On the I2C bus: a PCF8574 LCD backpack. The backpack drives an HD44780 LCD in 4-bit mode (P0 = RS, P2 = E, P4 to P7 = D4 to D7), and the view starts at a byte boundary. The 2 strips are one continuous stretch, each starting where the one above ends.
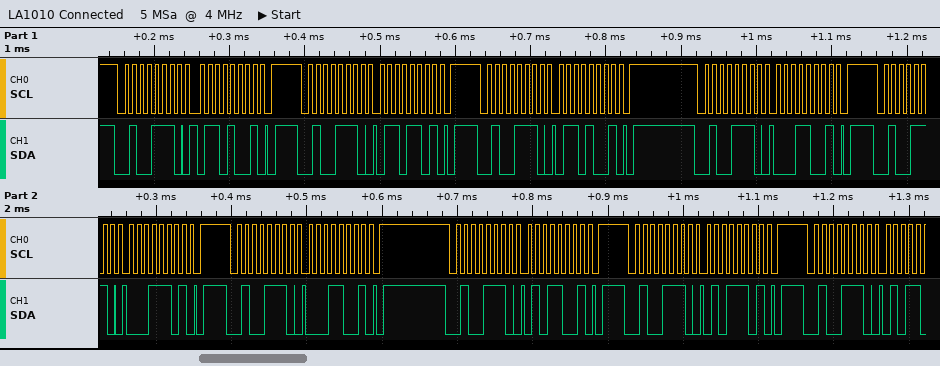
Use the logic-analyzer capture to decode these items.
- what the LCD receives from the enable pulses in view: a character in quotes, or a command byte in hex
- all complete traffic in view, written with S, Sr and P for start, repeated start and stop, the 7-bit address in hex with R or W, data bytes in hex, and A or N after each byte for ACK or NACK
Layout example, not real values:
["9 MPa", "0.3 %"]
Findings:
["'a'", "S 27W A 69 A P S 27W A 6D A P S 27W A 69 A P S 27W A 19 A P S 27W A 1D A P S 27W A 19 A P S 27W A 59 A P S 27W A 5D A P S 27W A"]
